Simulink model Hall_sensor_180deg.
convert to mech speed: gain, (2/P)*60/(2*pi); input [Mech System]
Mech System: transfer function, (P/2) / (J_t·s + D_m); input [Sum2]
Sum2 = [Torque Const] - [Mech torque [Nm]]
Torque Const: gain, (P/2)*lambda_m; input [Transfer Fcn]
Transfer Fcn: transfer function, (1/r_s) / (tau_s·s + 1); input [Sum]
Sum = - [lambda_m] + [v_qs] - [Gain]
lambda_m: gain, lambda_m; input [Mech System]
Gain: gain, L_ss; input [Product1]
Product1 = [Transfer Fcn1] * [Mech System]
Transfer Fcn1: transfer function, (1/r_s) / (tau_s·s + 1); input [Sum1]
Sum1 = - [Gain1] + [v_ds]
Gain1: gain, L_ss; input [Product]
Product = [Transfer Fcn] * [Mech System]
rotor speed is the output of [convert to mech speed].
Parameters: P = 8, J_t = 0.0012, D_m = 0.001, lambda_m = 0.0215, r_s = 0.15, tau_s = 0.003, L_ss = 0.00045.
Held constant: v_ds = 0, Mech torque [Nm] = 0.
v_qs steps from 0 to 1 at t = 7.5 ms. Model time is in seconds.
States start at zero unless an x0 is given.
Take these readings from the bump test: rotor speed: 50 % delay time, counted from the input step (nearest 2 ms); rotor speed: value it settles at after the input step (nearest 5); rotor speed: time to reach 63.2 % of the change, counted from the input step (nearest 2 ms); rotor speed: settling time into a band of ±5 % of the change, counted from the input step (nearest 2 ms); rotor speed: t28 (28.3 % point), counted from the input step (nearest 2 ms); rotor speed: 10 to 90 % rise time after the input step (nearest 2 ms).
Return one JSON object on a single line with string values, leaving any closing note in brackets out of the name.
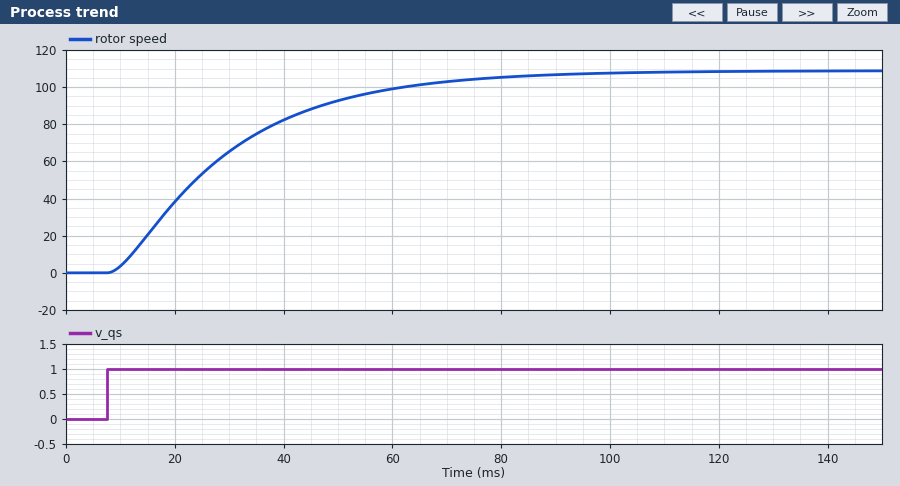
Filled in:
{"rotor speed: 50 % delay time, counted from the input step": "18 ms", "rotor speed: value it settles at after the input step": "110", "rotor speed: time to reach 63.2 % of the change, counted from the input step": "24 ms", "rotor speed: settling time into a band of ±5 % of the change, counted from the input step": "64 ms", "rotor speed: t28 (28.3 % point), counted from the input step": "10 ms", "rotor speed: 10 to 90 % rise time after the input step": "46 ms"}
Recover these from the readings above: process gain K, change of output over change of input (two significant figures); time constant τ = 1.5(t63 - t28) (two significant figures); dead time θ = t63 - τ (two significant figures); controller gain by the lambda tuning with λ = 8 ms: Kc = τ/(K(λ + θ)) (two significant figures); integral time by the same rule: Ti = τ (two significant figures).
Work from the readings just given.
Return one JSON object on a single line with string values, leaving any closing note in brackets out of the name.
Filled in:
{"process gain K, change of output over change of input": "110", "time constant τ = 1.5(t63 - t28)": "21 ms", "dead time θ = t63 - τ": "3.0 ms", "controller gain by the lambda tuning with λ = 8 ms: Kc = τ/(K(λ + θ))": "0.017", "integral time by the same rule: Ti = τ": "21 ms"}
